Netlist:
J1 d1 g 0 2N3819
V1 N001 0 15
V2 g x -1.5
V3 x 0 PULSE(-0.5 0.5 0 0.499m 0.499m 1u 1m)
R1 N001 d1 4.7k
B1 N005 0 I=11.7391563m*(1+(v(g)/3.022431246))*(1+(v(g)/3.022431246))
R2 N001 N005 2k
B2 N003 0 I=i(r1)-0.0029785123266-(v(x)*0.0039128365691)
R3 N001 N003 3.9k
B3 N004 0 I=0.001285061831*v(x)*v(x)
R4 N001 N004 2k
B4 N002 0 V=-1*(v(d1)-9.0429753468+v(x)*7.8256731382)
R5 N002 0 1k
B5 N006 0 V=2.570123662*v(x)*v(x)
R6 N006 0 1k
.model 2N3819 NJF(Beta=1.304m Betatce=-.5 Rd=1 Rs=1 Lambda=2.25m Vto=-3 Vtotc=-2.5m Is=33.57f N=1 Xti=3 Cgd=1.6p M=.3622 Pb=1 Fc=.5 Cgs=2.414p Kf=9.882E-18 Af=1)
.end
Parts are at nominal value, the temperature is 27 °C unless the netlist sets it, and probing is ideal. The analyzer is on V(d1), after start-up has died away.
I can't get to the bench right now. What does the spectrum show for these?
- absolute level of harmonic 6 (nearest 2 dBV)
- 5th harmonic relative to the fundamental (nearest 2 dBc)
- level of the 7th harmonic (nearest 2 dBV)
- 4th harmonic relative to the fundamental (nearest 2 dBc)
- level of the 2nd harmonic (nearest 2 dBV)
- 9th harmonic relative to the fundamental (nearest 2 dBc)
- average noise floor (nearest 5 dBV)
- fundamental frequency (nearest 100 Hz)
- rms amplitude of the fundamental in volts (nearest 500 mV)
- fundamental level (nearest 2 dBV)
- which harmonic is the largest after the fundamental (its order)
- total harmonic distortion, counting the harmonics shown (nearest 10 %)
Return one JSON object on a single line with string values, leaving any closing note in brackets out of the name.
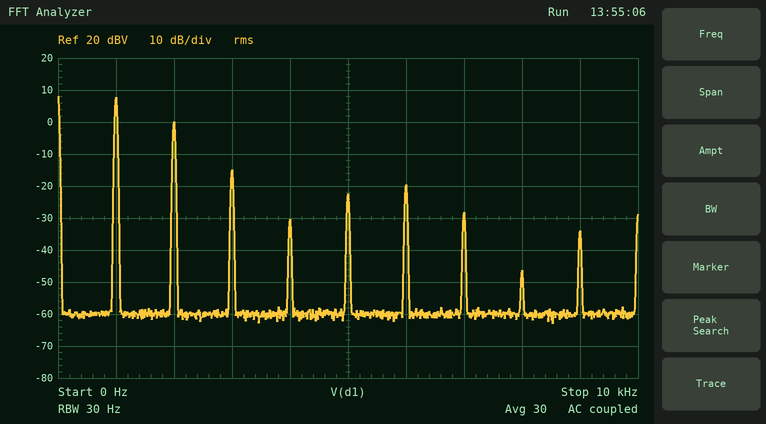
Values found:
{"absolute level of harmonic 6": "-20 dBV", "5th harmonic relative to the fundamental": "-30 dBc", "level of the 7th harmonic": "-28 dBV", "4th harmonic relative to the fundamental": "-38 dBc", "level of the 2nd harmonic": "0 dBV", "9th harmonic relative to the fundamental": "-42 dBc", "average noise floor": "-60 dBV", "fundamental frequency": "1.0 kHz", "rms amplitude of the fundamental in volts": "2.5 V", "fundamental level": "8 dBV", "which harmonic is the largest after the fundamental": "2", "total harmonic distortion, counting the harmonics shown": "40 %"}
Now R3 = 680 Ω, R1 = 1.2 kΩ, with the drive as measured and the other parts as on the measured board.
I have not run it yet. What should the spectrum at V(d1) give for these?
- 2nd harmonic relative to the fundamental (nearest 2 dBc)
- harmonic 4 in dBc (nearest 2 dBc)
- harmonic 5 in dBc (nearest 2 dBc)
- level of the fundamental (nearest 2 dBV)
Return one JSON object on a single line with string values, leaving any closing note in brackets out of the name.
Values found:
{"2nd harmonic relative to the fundamental": "-22 dBc", "harmonic 4 in dBc": "-34 dBc", "harmonic 5 in dBc": "-28 dBc", "level of the fundamental": "2 dBV"}
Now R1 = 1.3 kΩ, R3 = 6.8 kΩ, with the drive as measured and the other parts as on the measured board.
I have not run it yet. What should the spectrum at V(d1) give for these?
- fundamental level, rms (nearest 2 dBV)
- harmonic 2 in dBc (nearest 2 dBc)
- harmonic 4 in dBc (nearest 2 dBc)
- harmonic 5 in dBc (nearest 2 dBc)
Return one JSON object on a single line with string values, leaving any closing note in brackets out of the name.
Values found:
{"fundamental level, rms": "4 dBV", "harmonic 2 in dBc": "-22 dBc", "harmonic 4 in dBc": "-34 dBc", "harmonic 5 in dBc": "-28 dBc"}
